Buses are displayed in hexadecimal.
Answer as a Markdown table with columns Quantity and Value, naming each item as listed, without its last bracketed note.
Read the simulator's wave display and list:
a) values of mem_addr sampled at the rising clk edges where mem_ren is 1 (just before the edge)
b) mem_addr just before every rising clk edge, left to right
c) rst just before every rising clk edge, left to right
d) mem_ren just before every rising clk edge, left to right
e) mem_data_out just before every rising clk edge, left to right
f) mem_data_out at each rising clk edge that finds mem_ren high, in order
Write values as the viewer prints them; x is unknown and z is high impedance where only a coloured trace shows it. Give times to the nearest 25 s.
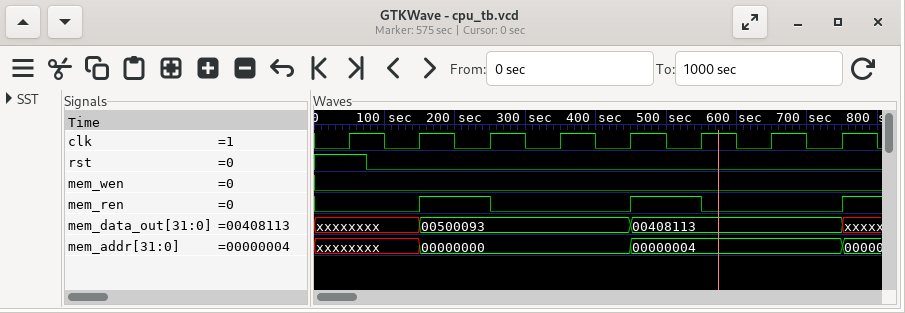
| Quantity | Value |
|---|---|
| values of mem_addr sampled at the rising clk edges where mem_ren is 1 | 00000000, 00000004 |
| mem_addr just before every rising clk edge, left to right | xxxxxxxx, xxxxxxxx, 00000000, 00000000, 00000000, 00000004, 00000004, 00000004 |
| rst just before every rising clk edge, left to right | 1 0 0 0 0 0 0 0 |
| mem_ren just before every rising clk edge, left to right | 0 0 1 0 0 1 0 0 |
| mem_data_out just before every rising clk edge, left to right | xxxxxxxx, xxxxxxxx, 00500093, 00500093, 00500093, 00408113, 00408113, 00408113 |
| mem_data_out at each rising clk edge that finds mem_ren high, in order | 00500093, 00408113 |
